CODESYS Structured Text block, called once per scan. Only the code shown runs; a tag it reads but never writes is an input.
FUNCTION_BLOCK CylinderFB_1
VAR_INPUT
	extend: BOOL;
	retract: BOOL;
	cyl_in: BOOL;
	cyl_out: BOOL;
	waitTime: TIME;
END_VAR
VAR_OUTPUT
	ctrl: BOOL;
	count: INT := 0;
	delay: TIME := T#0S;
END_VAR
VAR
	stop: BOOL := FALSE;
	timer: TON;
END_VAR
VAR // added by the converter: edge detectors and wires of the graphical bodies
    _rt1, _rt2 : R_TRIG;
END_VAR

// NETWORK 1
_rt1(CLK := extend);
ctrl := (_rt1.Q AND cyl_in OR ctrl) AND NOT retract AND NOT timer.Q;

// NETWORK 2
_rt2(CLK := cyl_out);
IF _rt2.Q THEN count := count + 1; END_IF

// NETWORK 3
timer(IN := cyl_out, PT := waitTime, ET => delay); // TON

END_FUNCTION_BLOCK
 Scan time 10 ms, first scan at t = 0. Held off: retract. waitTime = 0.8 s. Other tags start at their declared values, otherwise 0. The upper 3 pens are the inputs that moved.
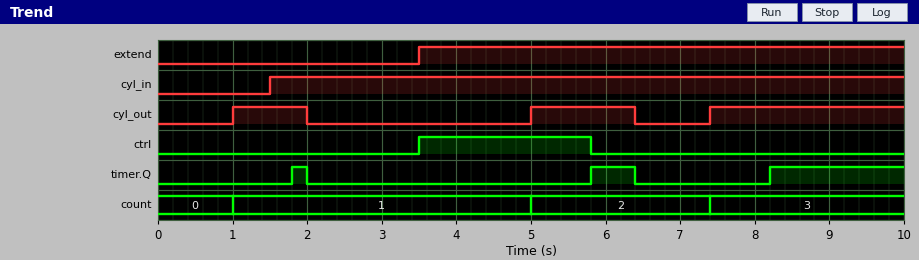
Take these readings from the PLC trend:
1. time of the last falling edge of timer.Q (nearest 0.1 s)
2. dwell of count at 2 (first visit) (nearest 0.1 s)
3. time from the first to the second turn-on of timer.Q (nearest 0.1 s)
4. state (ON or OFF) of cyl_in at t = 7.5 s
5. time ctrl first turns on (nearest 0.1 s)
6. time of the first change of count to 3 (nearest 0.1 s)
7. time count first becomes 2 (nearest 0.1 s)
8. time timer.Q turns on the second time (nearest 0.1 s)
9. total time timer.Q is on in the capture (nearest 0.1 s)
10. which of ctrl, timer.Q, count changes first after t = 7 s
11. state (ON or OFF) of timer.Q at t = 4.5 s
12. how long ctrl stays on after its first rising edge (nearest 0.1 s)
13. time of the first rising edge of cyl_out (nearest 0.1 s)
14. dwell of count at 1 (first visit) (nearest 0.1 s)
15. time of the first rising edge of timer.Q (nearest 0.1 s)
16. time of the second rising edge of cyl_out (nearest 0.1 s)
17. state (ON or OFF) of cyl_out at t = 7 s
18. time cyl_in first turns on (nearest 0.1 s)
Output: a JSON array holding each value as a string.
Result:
["6.4 s", "2.4 s", "4.0 s", "ON", "3.5 s", "7.4 s", "5.0 s", "5.8 s", "2.6 s", "count", "OFF", "2.3 s", "1.0 s", "4.0 s", "1.8 s", "5.0 s", "OFF", "1.5 s"]
